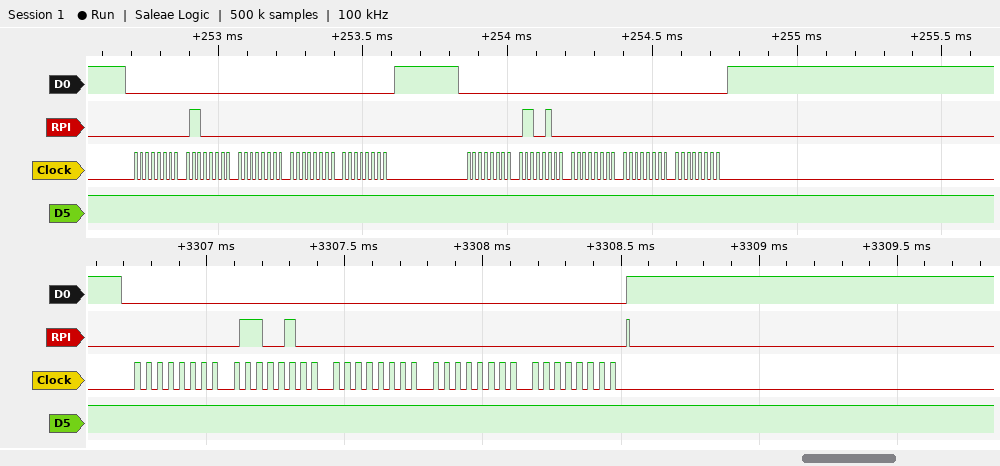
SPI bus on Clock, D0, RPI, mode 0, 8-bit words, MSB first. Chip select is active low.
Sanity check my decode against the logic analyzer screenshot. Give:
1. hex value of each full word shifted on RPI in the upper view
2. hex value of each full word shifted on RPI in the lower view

00, 60, 00, 00, 00, 00, 64, 00, 00, 00
00, 64, 00, 00, 00
